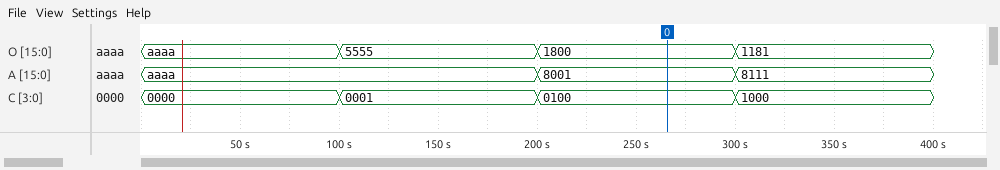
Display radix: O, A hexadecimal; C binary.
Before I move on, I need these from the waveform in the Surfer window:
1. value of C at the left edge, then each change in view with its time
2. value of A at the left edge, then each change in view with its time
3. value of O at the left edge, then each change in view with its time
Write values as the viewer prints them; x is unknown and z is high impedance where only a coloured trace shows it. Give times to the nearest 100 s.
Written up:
0000, 0001 at 100 s, 0100 at 200 s, 1000 at 300 s
aaaa, 8001 at 200 s, 8111 at 300 s
aaaa, 5555 at 100 s, 1800 at 200 s, 1181 at 300 s
